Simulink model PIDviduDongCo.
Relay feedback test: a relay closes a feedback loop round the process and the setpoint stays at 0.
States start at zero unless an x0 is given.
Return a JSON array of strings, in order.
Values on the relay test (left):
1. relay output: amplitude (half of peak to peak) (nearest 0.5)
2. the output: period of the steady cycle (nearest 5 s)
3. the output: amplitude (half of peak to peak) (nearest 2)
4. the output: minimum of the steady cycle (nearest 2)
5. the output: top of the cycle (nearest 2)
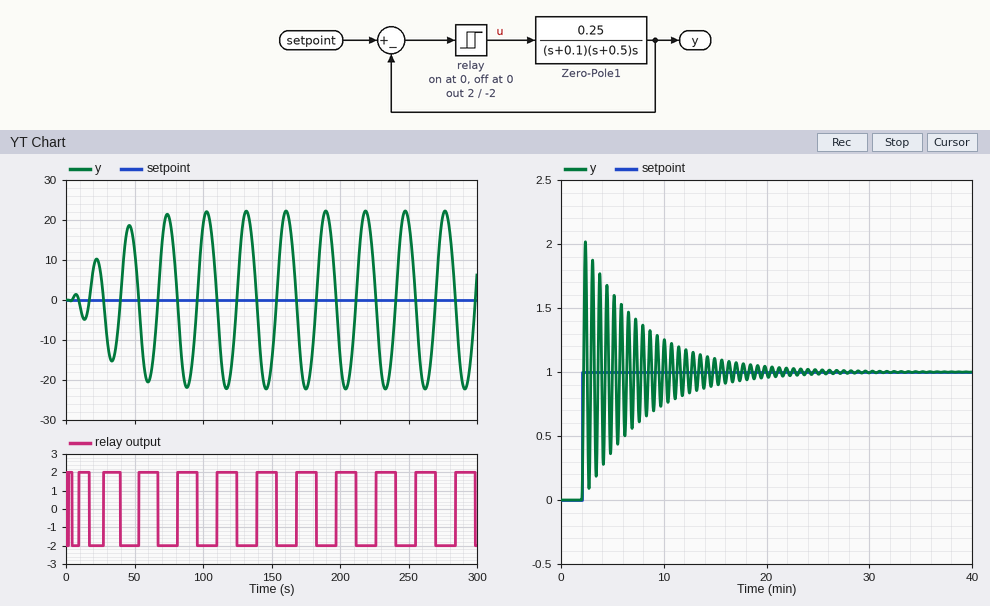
["2.0", "30 s", "22", "-22", "22"]
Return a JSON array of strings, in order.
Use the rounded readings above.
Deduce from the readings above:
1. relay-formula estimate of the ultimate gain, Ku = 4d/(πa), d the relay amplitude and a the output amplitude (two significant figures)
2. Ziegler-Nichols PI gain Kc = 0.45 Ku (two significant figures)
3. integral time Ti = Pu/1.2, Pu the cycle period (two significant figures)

["0.12", "0.054", "25 s"]
